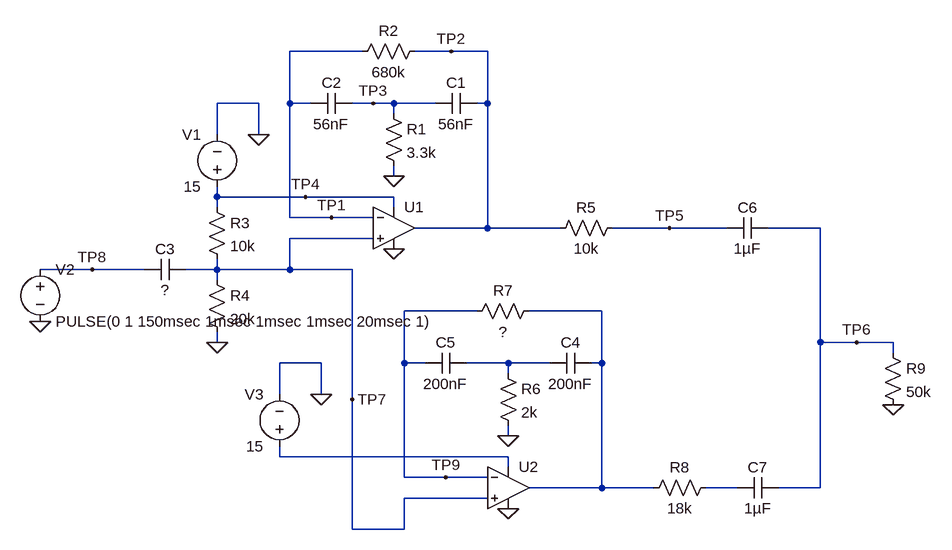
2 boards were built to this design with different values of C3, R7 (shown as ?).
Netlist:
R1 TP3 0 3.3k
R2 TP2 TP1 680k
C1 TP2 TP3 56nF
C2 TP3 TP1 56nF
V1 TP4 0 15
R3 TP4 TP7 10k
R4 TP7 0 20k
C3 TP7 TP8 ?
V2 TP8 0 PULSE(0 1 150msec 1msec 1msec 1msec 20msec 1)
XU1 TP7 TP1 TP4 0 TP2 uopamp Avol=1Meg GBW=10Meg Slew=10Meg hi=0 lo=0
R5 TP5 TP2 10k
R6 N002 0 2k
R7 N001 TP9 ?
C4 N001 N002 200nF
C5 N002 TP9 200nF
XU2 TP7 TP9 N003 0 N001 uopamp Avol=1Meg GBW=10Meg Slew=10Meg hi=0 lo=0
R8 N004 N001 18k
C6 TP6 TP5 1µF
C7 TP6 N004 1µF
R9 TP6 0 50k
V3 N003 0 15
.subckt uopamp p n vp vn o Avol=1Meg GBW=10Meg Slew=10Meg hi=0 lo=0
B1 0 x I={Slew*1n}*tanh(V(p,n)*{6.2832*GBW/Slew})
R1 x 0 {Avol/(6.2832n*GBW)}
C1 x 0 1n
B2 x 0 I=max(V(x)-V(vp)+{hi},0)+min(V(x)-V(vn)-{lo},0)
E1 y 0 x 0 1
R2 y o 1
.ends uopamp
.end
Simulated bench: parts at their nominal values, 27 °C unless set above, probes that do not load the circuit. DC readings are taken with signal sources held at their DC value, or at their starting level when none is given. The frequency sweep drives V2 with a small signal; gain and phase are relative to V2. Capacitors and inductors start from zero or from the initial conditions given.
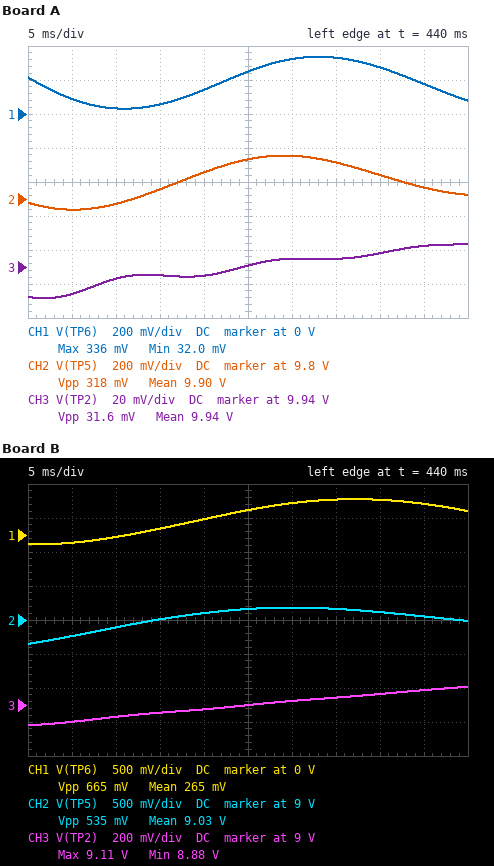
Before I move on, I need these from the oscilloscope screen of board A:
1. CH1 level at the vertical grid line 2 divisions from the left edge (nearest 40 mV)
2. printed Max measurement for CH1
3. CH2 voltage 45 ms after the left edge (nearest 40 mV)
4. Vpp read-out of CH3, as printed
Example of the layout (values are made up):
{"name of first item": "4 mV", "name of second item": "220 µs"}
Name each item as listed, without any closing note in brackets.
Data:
{"CH1 level at the vertical grid line 2 divisions from the left edge": "40 mV", "printed Max measurement for CH1": "336 mV", "CH2 voltage 45 ms after the left edge": "9.88 V", "Vpp read-out of CH3, as printed": "31.6 mV"}
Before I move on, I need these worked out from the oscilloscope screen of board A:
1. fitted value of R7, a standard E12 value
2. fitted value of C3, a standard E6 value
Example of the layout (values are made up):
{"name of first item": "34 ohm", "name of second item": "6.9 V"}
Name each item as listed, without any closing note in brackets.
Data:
{"fitted value of R7, a standard E12 value": "680 kΩ", "fitted value of C3, a standard E6 value": "15 µF"}
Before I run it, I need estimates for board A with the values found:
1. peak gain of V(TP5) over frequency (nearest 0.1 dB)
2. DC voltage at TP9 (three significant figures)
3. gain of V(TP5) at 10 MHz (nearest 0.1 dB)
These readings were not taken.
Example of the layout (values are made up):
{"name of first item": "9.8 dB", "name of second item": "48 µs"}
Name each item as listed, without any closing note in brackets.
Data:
{"peak gain of V(TP5) over frequency": "35.9 dB", "DC voltage at TP9": "10.0 V", "gain of V(TP5) at 10 MHz": "-4.1 dB"}
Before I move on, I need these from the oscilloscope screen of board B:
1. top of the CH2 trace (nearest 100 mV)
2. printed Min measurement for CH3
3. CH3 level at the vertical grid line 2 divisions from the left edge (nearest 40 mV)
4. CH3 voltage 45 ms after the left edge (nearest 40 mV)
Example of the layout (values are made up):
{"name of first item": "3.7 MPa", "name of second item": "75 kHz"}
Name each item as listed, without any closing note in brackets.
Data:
{"top of the CH2 trace": "9.2 V", "printed Min measurement for CH3": "8.88 V", "CH3 level at the vertical grid line 2 divisions from the left edge": "8.92 V", "CH3 voltage 45 ms after the left edge": "9.08 V"}
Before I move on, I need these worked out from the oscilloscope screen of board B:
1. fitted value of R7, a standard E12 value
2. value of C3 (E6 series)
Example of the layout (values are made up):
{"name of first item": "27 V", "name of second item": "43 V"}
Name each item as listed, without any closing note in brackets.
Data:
{"fitted value of R7, a standard E12 value": "1.8 MΩ", "value of C3": "33 µF"}
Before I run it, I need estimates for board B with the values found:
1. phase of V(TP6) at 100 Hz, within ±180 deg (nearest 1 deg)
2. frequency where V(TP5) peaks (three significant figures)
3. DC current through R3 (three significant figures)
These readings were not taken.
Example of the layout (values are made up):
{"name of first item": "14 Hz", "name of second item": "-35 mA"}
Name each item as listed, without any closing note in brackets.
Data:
{"phase of V(TP6) at 100 Hz, within ±180 deg": "-76 deg", "frequency where V(TP5) peaks": "13.3 Hz", "DC current through R3": "500 µA"}
